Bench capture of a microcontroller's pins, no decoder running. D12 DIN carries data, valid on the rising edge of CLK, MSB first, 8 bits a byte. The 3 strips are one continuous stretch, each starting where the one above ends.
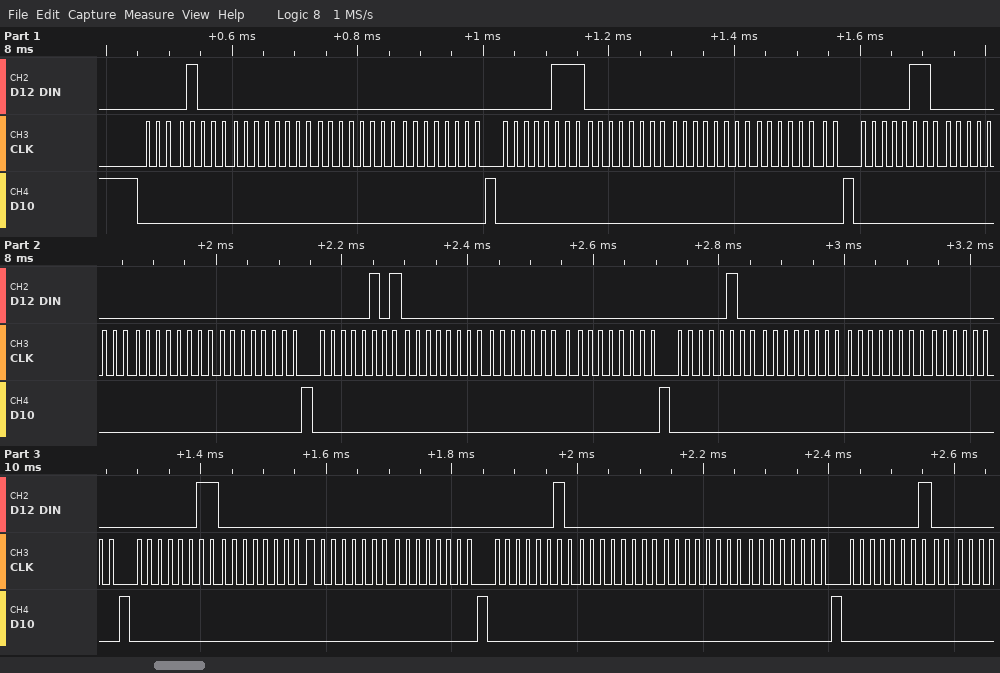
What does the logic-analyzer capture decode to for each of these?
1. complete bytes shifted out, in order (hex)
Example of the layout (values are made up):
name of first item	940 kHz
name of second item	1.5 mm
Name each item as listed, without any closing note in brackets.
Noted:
complete bytes shifted out, in order	0x08 0x00 0x00 0x00 0x07 0x00 0x00 0x00 0x06 0x00 0x00 0x00 0x05 0x00 0x00 0x00 0x04 0x00 0x00 0x00 0x03 0x00 0x00 0x00 0x02 0x00 0x00 0x00 0x01
